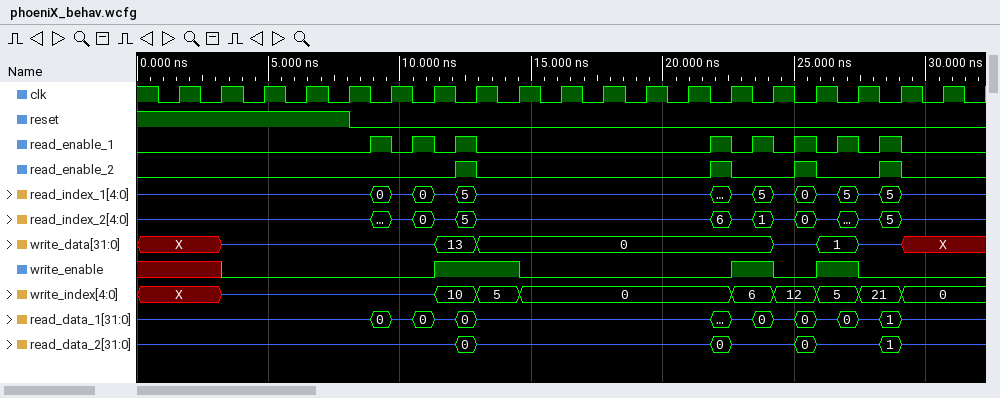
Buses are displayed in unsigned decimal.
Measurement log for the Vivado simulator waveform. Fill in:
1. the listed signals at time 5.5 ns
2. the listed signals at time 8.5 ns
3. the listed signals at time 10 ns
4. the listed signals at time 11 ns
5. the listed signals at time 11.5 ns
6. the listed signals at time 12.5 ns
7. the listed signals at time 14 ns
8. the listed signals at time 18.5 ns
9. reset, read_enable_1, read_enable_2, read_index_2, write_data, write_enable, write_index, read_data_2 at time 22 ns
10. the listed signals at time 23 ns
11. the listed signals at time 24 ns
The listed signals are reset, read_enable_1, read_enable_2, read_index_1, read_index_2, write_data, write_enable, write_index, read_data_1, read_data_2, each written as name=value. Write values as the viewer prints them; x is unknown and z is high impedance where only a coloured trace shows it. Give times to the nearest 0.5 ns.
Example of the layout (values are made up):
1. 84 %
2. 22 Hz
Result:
1. reset=1, read_enable_1=0, read_enable_2=0, read_index_1=z, read_index_2=z, write_data=z, write_enable=0, write_index=z, read_data_1=z, read_data_2=z
2. reset=0, read_enable_1=0, read_enable_2=0, read_index_1=z, read_index_2=z, write_data=z, write_enable=0, write_index=z, read_data_1=z, read_data_2=z
3. reset=0, read_enable_1=0, read_enable_2=0, read_index_1=z, read_index_2=z, write_data=z, write_enable=0, write_index=z, read_data_1=z, read_data_2=z
4. reset=0, read_enable_1=1, read_enable_2=0, read_index_1=0, read_index_2=0, write_data=z, write_enable=0, write_index=z, read_data_1=0, read_data_2=z
5. reset=0, read_enable_1=0, read_enable_2=0, read_index_1=z, read_index_2=z, write_data=13, write_enable=1, write_index=10, read_data_1=z, read_data_2=z
6. reset=0, read_enable_1=1, read_enable_2=1, read_index_1=5, read_index_2=5, write_data=13, write_enable=1, write_index=10, read_data_1=0, read_data_2=0
7. reset=0, read_enable_1=0, read_enable_2=0, read_index_1=z, read_index_2=z, write_data=0, write_enable=1, write_index=5, read_data_1=z, read_data_2=z
8. reset=0, read_enable_1=0, read_enable_2=0, read_index_1=z, read_index_2=z, write_data=0, write_enable=0, write_index=0, read_data_1=z, read_data_2=z
9. reset=0, read_enable_1=1, read_enable_2=1, read_index_2=6, write_data=0, write_enable=0, write_index=0, read_data_2=0
10. reset=0, read_enable_1=0, read_enable_2=0, read_index_1=z, read_index_2=z, write_data=0, write_enable=1, write_index=6, read_data_1=z, read_data_2=z
11. reset=0, read_enable_1=1, read_enable_2=0, read_index_1=5, read_index_2=1, write_data=0, write_enable=1, write_index=6, read_data_1=0, read_data_2=z
